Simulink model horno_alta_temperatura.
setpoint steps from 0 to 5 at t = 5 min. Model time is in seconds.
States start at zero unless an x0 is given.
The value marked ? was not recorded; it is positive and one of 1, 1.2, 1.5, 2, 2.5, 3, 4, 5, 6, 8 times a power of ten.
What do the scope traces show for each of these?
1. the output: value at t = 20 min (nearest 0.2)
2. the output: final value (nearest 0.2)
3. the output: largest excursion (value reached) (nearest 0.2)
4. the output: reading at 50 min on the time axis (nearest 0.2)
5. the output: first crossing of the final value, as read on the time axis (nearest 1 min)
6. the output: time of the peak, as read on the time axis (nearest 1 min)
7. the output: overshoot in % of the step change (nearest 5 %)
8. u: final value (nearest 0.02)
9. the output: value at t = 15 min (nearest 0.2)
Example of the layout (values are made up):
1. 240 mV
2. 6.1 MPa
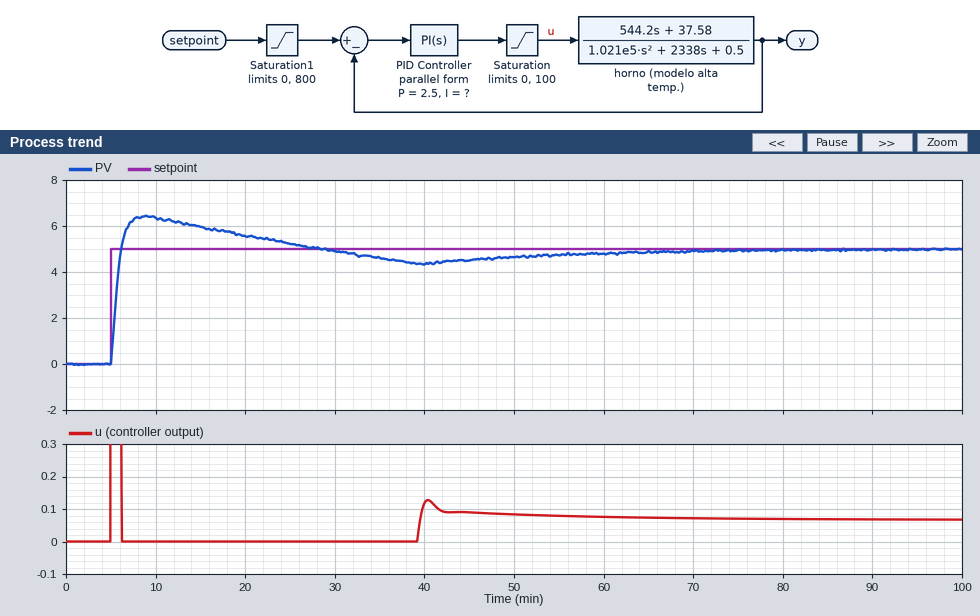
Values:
1. 5.6
2. 5.0
3. 6.4
4. 4.6
5. 6 min
6. 9 min
7. 30 %
8. 0.06
9. 6.0
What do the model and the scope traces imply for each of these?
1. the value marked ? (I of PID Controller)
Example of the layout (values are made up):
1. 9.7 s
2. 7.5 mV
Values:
1. 0.0025
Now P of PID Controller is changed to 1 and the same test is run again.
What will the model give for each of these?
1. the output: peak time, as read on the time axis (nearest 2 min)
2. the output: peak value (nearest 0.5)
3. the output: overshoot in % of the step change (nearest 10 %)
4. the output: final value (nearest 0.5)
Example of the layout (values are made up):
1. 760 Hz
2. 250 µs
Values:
1. 10 min
2. 6.0
3. 20 %
4. 5.0
